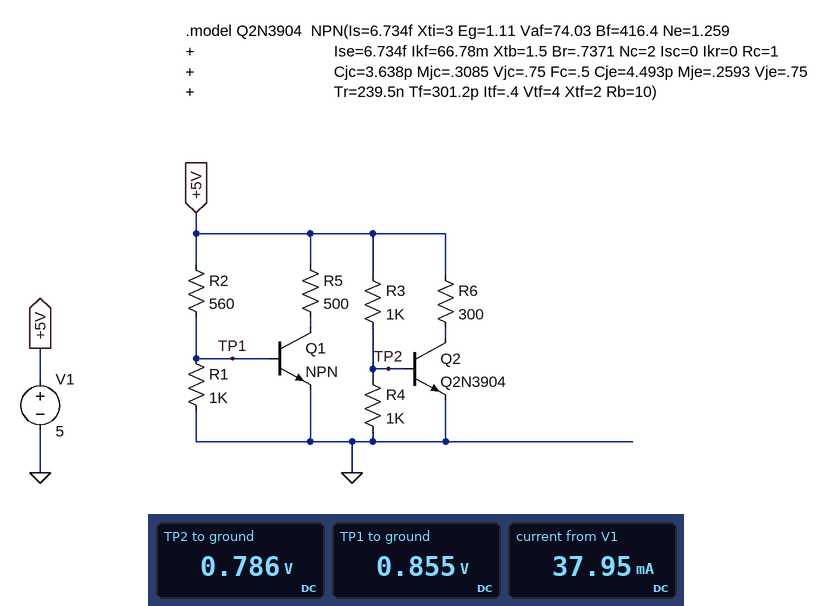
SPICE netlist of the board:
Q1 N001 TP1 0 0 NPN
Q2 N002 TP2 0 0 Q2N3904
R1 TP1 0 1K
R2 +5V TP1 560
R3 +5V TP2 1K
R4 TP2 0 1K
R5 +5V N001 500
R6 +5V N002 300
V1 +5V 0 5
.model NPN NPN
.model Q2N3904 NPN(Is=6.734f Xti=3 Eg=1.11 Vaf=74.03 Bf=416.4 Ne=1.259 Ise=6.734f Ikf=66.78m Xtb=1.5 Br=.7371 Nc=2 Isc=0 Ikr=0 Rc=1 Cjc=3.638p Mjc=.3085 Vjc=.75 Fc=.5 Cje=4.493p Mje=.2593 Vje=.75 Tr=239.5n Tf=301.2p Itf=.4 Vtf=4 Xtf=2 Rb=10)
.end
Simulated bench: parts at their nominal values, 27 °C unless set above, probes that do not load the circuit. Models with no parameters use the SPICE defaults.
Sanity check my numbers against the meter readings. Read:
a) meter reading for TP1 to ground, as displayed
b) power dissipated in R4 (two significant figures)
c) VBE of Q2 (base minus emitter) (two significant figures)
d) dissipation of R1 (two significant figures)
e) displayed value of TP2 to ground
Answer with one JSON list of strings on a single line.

["0.855 V", "620 µW", "790 mV", "730 µW", "0.786 V"]
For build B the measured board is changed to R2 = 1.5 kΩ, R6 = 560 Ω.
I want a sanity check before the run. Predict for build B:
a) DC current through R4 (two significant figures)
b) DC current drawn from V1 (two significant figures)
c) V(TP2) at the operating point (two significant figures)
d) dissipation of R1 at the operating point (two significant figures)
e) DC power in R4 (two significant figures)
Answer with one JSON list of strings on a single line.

["770 µA", "26 mA", "770 mV", "710 µW", "600 µW"]
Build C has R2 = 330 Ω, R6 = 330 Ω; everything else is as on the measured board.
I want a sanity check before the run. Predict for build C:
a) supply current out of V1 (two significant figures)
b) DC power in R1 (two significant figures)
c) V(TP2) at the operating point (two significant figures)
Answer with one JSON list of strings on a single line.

["42 mA", "750 µW", "780 mV"]
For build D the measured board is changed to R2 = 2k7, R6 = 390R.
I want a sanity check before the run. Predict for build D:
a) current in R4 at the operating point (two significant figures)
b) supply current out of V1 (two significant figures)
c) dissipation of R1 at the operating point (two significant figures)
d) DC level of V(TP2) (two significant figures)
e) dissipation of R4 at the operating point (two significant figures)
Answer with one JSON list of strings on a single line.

["780 µA", "28 mA", "700 µW", "780 mV", "610 µW"]
